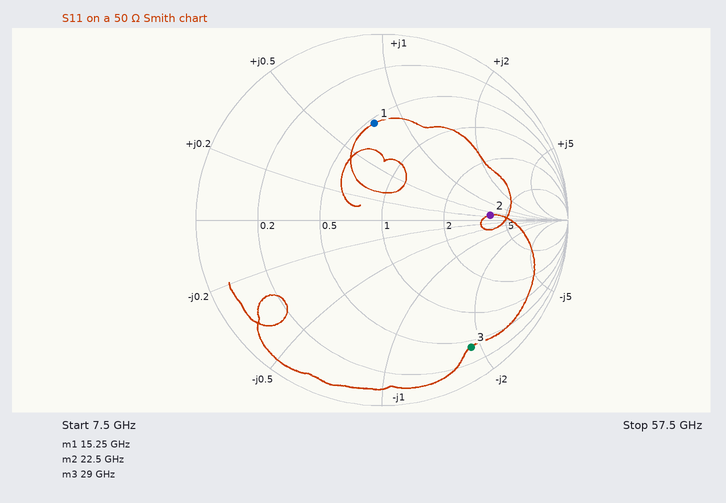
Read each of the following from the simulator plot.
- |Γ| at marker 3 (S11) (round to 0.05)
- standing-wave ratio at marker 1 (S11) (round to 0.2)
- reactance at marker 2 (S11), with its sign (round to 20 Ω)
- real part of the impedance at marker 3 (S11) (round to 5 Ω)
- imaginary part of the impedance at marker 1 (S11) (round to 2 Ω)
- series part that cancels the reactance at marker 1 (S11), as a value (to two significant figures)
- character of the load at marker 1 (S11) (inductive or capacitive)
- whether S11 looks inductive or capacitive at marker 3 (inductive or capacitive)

0.85
3.2
+20 Ω
20 Ω
+38 Ω
270 fF
inductive
capacitive
